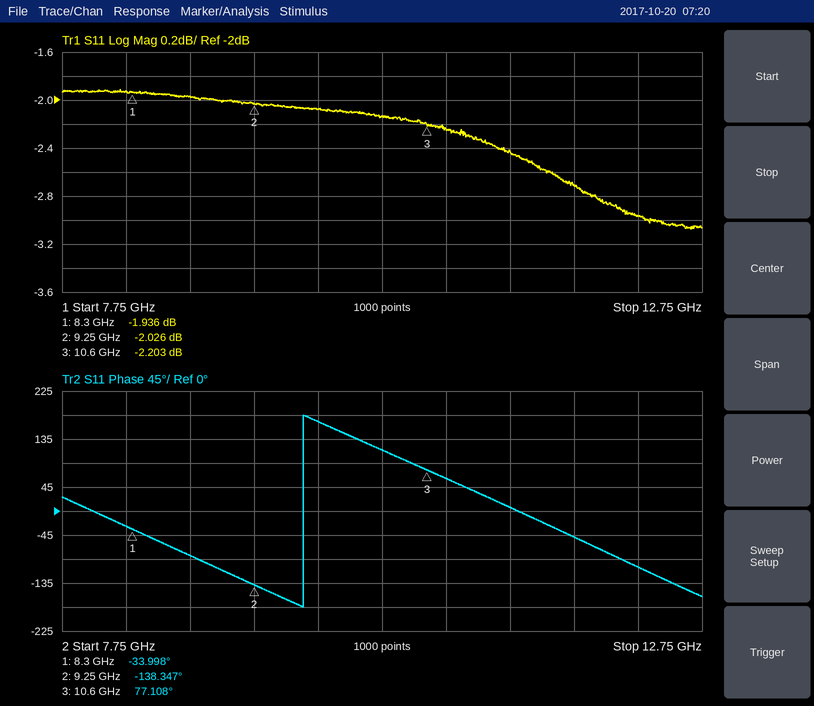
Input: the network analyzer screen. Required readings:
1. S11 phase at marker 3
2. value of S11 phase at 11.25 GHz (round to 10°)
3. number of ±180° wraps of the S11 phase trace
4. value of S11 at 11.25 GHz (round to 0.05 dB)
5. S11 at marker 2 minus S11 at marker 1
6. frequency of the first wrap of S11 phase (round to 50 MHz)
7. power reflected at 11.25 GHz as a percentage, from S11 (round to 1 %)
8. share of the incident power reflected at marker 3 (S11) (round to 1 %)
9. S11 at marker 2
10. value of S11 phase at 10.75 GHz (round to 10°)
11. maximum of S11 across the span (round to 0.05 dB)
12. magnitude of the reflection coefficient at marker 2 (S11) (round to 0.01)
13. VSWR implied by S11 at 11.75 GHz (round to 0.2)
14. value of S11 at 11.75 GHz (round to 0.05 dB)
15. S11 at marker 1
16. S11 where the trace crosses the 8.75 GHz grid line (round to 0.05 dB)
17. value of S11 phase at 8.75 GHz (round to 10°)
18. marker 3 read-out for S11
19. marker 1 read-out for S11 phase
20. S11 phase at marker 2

77.108°
10°
1
-2.45 dB
-0.090 dB
9.65 GHz
57 %
60 %
-2.026 dB
60°
-1.90 dB
0.79
6.4
-2.70 dB
-1.936 dB
-1.95 dB
-80°
-2.203 dB
-33.998°
-138.347°
